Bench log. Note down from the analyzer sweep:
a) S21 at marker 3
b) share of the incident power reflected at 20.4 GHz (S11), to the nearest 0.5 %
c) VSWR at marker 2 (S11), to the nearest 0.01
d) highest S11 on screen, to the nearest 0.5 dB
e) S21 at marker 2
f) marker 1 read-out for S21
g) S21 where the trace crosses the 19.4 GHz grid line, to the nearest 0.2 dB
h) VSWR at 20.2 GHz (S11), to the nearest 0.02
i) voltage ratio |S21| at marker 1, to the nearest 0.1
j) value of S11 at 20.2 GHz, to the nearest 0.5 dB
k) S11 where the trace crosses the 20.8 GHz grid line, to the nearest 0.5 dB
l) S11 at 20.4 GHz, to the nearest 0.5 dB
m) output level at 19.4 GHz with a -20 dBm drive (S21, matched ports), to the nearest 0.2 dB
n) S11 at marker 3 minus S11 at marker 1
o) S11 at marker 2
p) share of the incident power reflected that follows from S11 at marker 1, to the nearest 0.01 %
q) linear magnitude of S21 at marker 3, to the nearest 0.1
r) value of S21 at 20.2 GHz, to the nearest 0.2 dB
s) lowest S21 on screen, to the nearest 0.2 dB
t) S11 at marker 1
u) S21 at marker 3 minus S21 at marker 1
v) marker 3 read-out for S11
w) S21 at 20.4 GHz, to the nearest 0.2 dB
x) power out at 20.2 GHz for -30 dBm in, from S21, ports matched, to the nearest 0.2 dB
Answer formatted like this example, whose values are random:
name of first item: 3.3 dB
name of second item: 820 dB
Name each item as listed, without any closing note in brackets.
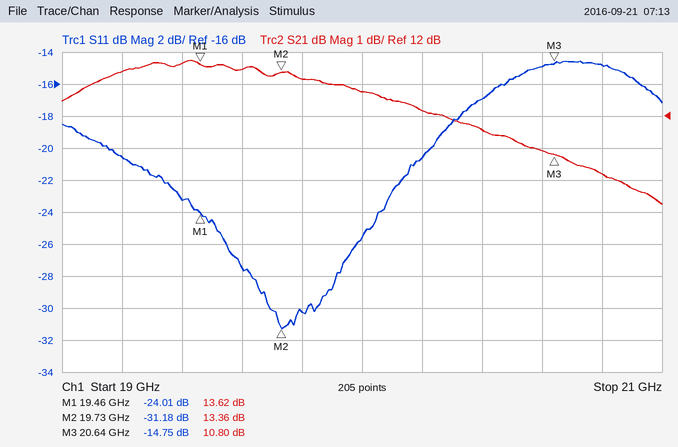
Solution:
S21 at marker 3: 10.80 dB
share of the incident power reflected at 20.4 GHz (S11), to the nearest 0.5 %: 2.0 %
VSWR at marker 2 (S11), to the nearest 0.01: 1.06
highest S11 on screen, to the nearest 0.5 dB: -14.5 dB
S21 at marker 2: 13.36 dB
marker 1 read-out for S21: 13.62 dB
S21 where the trace crosses the 19.4 GHz grid line, to the nearest 0.2 dB: 13.6 dB
VSWR at 20.2 GHz (S11), to the nearest 0.02: 1.20
voltage ratio |S21| at marker 1, to the nearest 0.1: 4.8
value of S11 at 20.2 GHz, to the nearest 0.5 dB: -20.5 dB
S11 where the trace crosses the 20.8 GHz grid line, to the nearest 0.5 dB: -15.0 dB
S11 at 20.4 GHz, to the nearest 0.5 dB: -17.0 dB
output level at 19.4 GHz with a -20 dBm drive (S21, matched ports), to the nearest 0.2 dB: -6.4 dBm
S11 at marker 3 minus S11 at marker 1: 9.26 dB
S11 at marker 2: -31.18 dB
share of the incident power reflected that follows from S11 at marker 1, to the nearest 0.01 %: 0.40 %
linear magnitude of S21 at marker 3, to the nearest 0.1: 3.5
value of S21 at 20.2 GHz, to the nearest 0.2 dB: 12.2 dB
lowest S21 on screen, to the nearest 0.2 dB: 9.2 dB
S11 at marker 1: -24.01 dB
S21 at marker 3 minus S21 at marker 1: -2.82 dB
marker 3 read-out for S11: -14.75 dB
S21 at 20.4 GHz, to the nearest 0.2 dB: 11.6 dB
power out at 20.2 GHz for -30 dBm in, from S21, ports matched, to the nearest 0.2 dB: -17.8 dBm
